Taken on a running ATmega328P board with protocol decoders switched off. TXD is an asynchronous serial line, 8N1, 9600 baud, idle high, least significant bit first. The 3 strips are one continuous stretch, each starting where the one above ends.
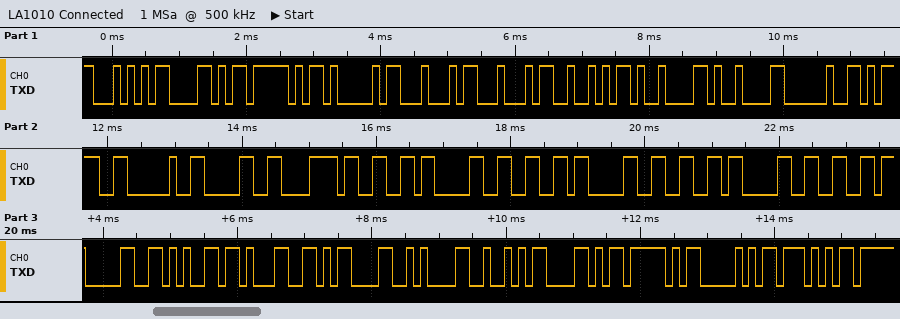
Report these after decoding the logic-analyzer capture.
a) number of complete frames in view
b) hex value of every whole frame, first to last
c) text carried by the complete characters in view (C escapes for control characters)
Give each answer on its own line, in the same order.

31
0x54 0x58 0x5F 0x41 0x44 0x44 0x52 0x09 0x09 0x20 0x3D 0x20 0x30 0x78 0x66 0x30 0x66 0x30 0x66 0x30 0x66 0x30 0x65 0x31 0x0D 0x0A 0x52 0x58 0x5F 0x50 0x57
"TX_ADDR\t\t = 0xf0f0f0f0e1\r\nRX_PW"
